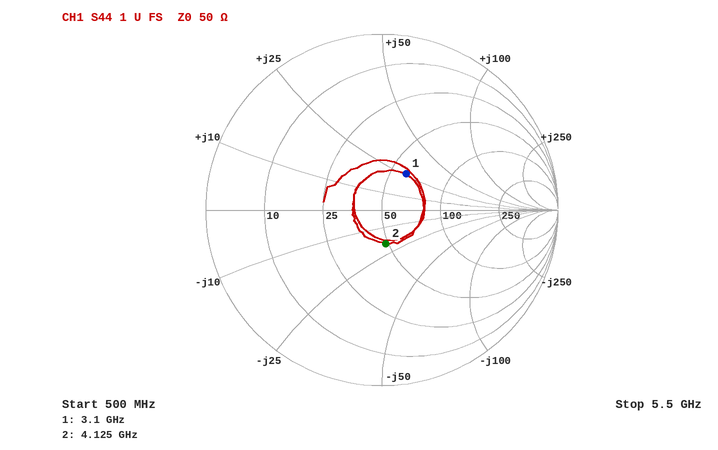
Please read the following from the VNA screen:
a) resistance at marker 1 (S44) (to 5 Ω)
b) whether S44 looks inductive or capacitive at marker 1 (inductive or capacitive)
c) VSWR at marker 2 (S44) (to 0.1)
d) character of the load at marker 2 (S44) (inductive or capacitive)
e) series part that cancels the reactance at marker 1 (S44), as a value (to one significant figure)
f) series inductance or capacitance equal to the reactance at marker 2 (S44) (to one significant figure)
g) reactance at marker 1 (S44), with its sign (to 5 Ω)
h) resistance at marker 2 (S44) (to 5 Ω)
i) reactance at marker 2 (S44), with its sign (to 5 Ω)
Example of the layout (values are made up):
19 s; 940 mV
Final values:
60 Ω; inductive; 1.5; capacitive; 2 pF; 2 pF; +25 Ω; 50 Ω; -20 Ω
